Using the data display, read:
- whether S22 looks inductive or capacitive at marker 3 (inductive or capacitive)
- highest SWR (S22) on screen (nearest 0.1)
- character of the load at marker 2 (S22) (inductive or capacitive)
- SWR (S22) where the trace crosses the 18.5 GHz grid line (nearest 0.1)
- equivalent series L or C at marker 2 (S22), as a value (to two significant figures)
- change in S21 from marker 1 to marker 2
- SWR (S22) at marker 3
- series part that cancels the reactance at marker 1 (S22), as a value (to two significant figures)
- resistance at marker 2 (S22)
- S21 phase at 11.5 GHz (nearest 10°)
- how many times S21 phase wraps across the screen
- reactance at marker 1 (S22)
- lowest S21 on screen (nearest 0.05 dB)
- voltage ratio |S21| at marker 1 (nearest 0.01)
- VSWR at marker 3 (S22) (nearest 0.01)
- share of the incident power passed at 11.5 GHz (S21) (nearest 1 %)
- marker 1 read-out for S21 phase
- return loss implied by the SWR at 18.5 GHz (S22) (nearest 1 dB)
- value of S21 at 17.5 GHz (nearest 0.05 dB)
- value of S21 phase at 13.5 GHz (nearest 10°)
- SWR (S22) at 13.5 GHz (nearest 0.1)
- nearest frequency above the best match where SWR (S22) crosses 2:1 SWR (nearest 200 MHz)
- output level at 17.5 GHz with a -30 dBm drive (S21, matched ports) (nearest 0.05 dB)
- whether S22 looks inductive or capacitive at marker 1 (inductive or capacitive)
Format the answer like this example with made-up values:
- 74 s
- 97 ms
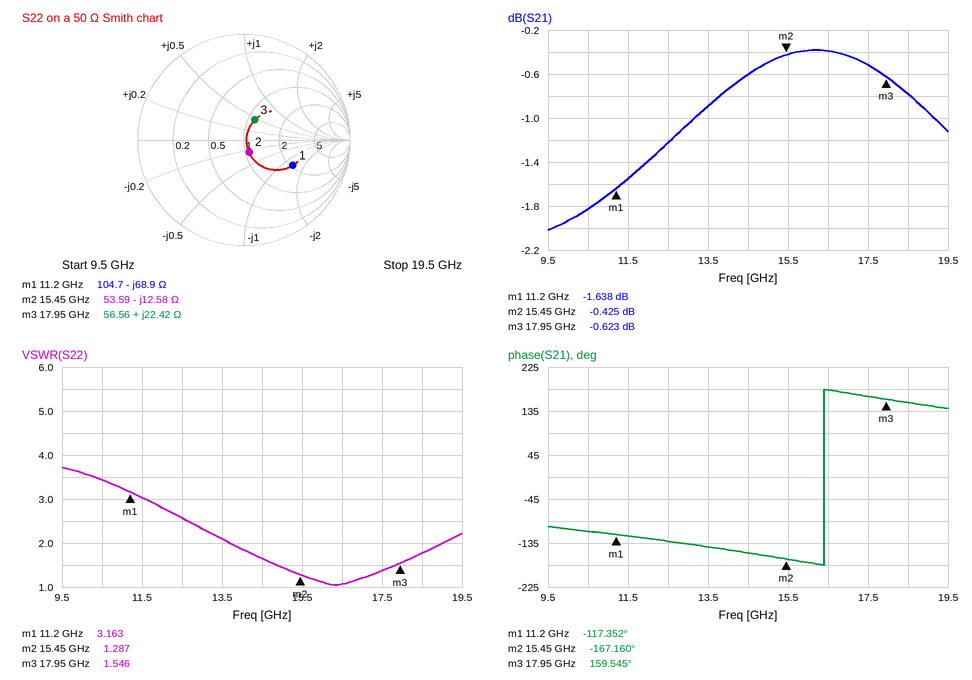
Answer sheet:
- inductive
- 3.7
- capacitive
- 1.8
- 820 fF
- 1.213 dB
- 1.546
- 980 pH
- 53.59 Ω
- -120°
- 1
- -68.9 Ω
- -2.00 dB
- 0.83
- 1.55
- 70 %
- -117.352°
- 11 dB
- -0.50 dB
- -140°
- 2.1
- 19.0 GHz
- -30.50 dBm
- capacitive
